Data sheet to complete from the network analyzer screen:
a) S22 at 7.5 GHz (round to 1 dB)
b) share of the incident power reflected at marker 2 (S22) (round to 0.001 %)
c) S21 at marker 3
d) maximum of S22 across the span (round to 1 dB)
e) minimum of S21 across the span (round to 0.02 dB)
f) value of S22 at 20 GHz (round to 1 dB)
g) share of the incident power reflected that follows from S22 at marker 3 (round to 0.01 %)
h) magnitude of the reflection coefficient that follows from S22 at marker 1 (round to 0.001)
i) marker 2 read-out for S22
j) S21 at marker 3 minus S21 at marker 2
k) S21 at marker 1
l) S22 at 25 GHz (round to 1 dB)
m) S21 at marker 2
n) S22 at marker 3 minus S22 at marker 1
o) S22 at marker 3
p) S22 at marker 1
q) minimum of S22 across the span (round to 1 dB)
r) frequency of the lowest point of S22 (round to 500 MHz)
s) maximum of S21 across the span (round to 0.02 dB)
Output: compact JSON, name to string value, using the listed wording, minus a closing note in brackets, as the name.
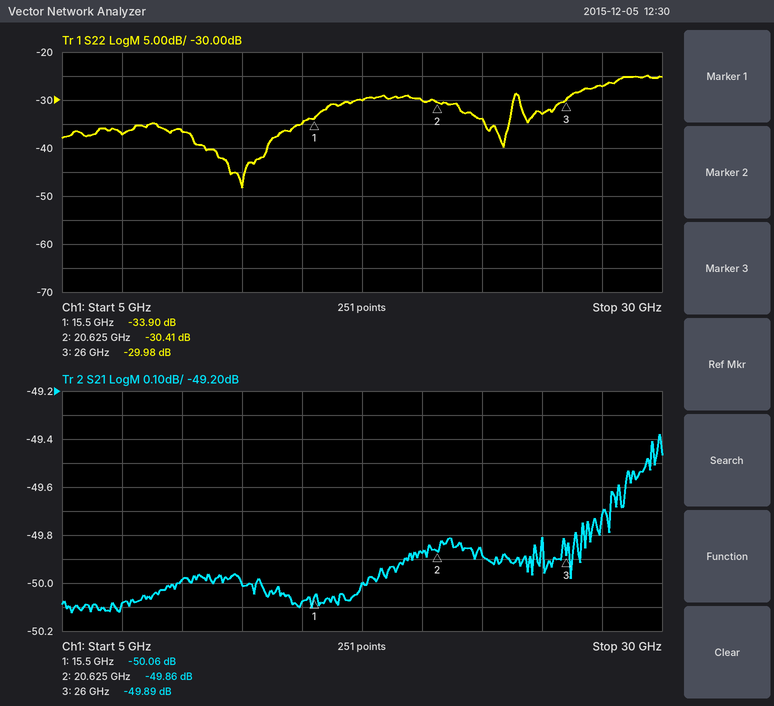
{"S22 at 7.5 GHz": "-37 dB", "share of the incident power reflected at marker 2 (S22)": "0.091 %", "S21 at marker 3": "-49.89 dB", "maximum of S22 across the span": "-25 dB", "minimum of S21 across the span": "-50.12 dB", "value of S22 at 20 GHz": "-30 dB", "share of the incident power reflected that follows from S22 at marker 3": "0.10 %", "magnitude of the reflection coefficient that follows from S22 at marker 1": "0.020", "marker 2 read-out for S22": "-30.41 dB", "S21 at marker 3 minus S21 at marker 2": "-0.03 dB", "S21 at marker 1": "-50.06 dB", "S22 at 25 GHz": "-33 dB", "S21 at marker 2": "-49.86 dB", "S22 at marker 3 minus S22 at marker 1": "3.92 dB", "S22 at marker 3": "-29.98 dB", "S22 at marker 1": "-33.90 dB", "minimum of S22 across the span": "-48 dB", "frequency of the lowest point of S22": "12.5 GHz", "maximum of S21 across the span": "-49.38 dB"}
